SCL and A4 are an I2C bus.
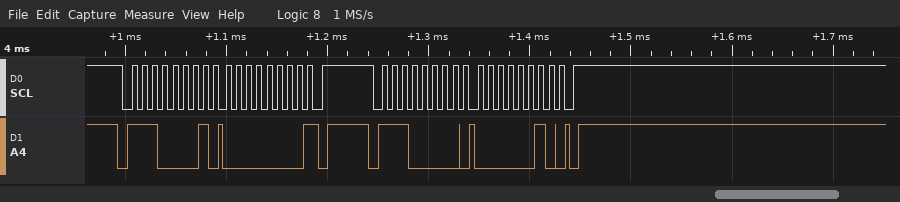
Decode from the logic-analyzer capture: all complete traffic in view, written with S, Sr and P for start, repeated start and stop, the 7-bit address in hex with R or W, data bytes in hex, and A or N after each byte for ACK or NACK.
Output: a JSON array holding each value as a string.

["S 70R A 00 N P S 70W A 02 A P"]
